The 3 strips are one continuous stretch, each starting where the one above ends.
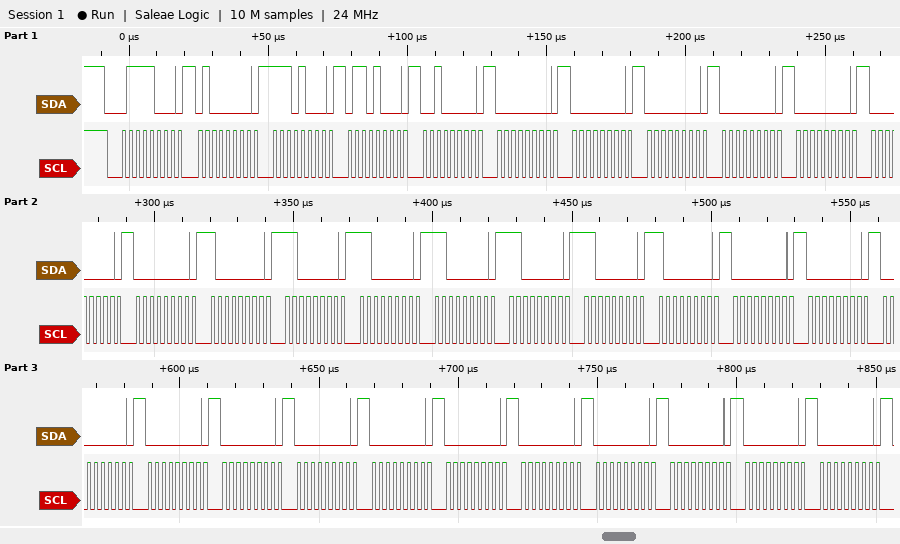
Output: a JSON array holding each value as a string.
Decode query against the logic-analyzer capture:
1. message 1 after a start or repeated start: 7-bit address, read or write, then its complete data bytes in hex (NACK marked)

["0x3C write: 40 E8 68 20 00 00 00 00 00 00 00 80 C0 C0 C0 C0 C0 80 00 00 00 00 00 00 00 00 00 00 00 00 00"]
